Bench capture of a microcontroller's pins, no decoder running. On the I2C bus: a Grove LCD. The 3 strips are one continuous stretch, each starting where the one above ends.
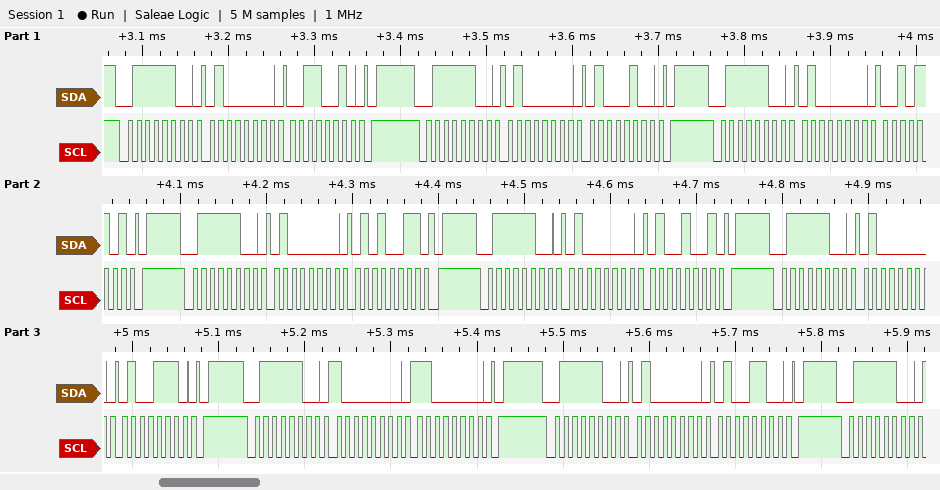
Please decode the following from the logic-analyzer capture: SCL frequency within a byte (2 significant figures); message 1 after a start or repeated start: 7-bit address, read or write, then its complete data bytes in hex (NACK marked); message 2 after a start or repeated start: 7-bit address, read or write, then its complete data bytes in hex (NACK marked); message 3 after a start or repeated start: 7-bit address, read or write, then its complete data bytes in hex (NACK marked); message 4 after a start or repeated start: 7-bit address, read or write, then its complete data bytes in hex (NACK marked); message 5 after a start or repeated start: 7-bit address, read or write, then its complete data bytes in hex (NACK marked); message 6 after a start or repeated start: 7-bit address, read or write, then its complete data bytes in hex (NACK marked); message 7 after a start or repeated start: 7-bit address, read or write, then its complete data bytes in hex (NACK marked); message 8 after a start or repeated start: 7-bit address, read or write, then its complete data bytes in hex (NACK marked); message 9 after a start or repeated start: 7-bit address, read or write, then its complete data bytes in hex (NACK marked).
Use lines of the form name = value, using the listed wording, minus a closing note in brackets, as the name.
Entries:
SCL frequency within a byte = 100 kHz
message 1 after a start or repeated start: 7-bit address, read or write, then its complete data bytes in hex = 0x3E write: 40 32
message 2 after a start or repeated start: 7-bit address, read or write, then its complete data bytes in hex = 0x3E write: 40 44
message 3 after a start or repeated start: 7-bit address, read or write, then its complete data bytes in hex = 0x3E write: 40 2D
message 4 after a start or repeated start: 7-bit address, read or write, then its complete data bytes in hex = 0x3E write: 40 53
message 5 after a start or repeated start: 7-bit address, read or write, then its complete data bytes in hex = 0x3E write: 40 49
message 6 after a start or repeated start: 7-bit address, read or write, then its complete data bytes in hex = 0x3E write: 40 4E
message 7 after a start or repeated start: 7-bit address, read or write, then its complete data bytes in hex = 0x3E write: 80 C0
message 8 after a start or repeated start: 7-bit address, read or write, then its complete data bytes in hex = 0x3E write: 40 4C
message 9 after a start or repeated start: 7-bit address, read or write, then its complete data bytes in hex = 0x3E write
